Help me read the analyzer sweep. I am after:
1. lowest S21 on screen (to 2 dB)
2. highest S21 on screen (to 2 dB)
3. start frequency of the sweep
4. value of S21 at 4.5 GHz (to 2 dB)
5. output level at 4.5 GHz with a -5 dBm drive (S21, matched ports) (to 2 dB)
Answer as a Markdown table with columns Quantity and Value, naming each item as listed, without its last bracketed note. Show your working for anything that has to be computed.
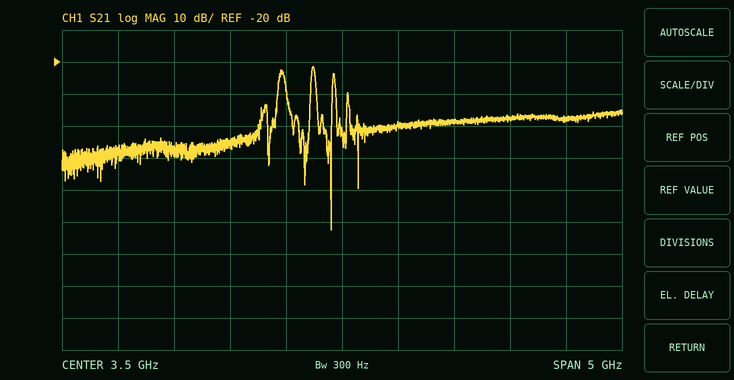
| Quantity | Value |
|---|---|
| lowest S21 on screen | -72 dB |
| highest S21 on screen | -22 dB |
| start frequency of the sweep | 1 GHz |
| value of S21 at 4.5 GHz | -38 dB |
| output level at 4.5 GHz with a -5 dBm drive (S21, matched ports) | -5 dBm + (-38 dB) = -44 dBm |
